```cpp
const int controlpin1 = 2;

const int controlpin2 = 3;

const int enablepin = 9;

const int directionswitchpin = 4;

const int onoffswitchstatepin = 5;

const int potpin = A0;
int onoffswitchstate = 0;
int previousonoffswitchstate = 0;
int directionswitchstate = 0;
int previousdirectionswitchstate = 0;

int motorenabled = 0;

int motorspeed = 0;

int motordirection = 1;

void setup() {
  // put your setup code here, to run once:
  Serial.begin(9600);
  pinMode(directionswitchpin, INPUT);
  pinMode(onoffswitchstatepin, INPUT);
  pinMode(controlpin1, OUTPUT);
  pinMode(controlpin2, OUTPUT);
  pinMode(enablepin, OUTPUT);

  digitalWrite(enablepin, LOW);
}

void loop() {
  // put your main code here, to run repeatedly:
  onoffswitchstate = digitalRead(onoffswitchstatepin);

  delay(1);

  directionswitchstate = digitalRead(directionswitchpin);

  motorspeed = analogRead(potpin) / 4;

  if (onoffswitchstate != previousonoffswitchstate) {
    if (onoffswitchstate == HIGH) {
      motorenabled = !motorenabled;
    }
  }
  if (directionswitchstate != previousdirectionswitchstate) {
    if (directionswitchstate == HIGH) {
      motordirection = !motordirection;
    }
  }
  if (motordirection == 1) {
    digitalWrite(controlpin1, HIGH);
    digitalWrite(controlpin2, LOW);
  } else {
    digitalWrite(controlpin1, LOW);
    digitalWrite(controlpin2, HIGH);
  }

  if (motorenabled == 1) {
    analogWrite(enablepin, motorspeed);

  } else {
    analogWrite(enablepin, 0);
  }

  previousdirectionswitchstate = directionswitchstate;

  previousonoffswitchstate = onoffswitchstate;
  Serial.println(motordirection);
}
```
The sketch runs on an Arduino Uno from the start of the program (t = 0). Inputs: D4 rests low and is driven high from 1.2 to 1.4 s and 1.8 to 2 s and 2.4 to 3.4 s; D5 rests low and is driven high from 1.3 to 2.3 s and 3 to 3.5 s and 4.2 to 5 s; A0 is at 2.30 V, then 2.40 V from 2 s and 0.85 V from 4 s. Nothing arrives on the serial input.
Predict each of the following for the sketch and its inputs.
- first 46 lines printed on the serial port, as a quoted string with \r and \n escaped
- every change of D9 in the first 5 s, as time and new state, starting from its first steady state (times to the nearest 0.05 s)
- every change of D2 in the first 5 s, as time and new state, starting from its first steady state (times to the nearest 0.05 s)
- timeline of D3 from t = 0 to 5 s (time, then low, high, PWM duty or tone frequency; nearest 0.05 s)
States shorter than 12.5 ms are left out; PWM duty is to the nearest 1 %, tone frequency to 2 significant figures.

"1\r\n1\r\n1\r\n1\r\n1\r\n1\r\n1\r\n1\r\n1\r\n1\r\n1\r\n1\r\n1\r\n1\r\n1\r\n1\r\n1\r\n1\r\n1\r\n1\r\n1\r\n1\r\n1\r\n1\r\n1\r\n1\r\n1\r\n1\r\n1\r\n1\r\n1\r\n1\r\n1\r\n1\r\n1\r\n1\r\n1\r\n1\r\n1\r\n1\r\n1\r\n1\r\n1\r\n1\r\n1\r\n1\r\n"
0 s low; 1.3 s PWM 46 %; 2 s PWM 48 %; 3 s low; 4.2 s PWM 17 %
0 s high; 1.2 s low; 1.8 s high; 2.4 s low
0 s low; 1.2 s high; 1.8 s low; 2.4 s high
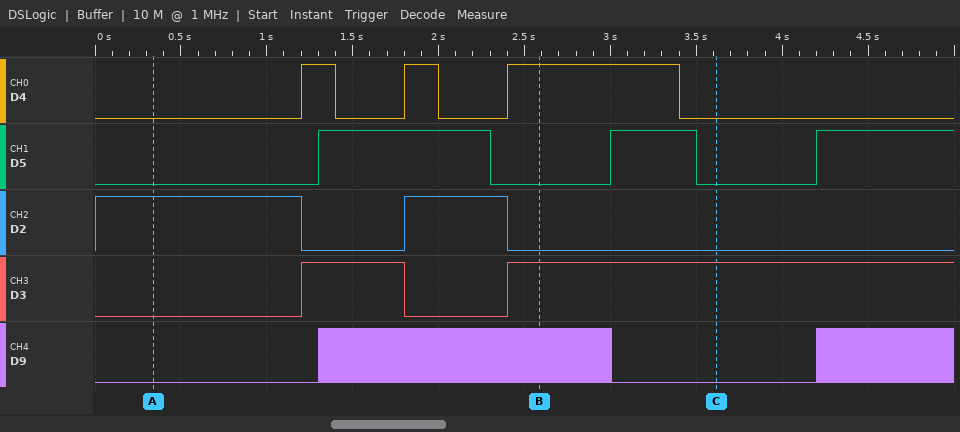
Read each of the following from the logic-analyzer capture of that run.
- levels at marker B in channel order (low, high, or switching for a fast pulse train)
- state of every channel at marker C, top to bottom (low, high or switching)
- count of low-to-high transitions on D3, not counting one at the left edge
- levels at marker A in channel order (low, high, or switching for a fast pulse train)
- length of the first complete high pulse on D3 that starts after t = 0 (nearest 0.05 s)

D4 high, D5 low, D2 low, D3 high, D9 switching
D4 low, D5 low, D2 low, D3 high, D9 low
2
D4 low, D5 low, D2 high, D3 low, D9 low
0.60 s
